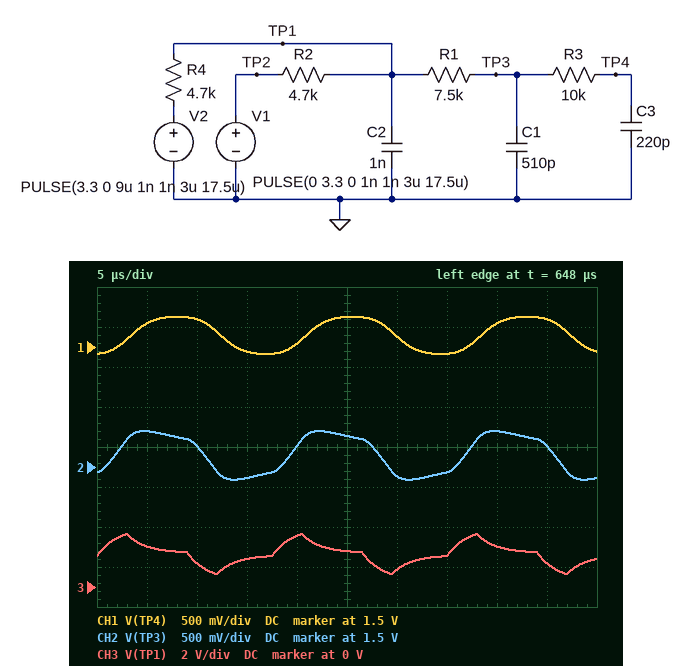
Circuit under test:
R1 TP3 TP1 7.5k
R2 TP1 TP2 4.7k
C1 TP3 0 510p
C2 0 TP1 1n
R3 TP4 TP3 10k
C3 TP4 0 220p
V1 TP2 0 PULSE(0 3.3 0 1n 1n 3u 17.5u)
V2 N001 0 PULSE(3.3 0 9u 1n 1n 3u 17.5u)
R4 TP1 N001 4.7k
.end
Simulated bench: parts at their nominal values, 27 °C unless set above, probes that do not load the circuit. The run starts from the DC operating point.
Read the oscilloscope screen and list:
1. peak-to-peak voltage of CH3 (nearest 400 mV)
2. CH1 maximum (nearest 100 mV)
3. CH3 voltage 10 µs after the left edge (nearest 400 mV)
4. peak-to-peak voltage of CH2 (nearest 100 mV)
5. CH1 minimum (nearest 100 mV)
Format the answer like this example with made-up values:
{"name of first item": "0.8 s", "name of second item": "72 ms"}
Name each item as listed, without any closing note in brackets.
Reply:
{"peak-to-peak voltage of CH3": "2.0 V", "CH1 maximum": "1.9 V", "CH3 voltage 10 µs after the left edge": "1.2 V", "peak-to-peak voltage of CH2": "600 mV", "CH1 minimum": "1.4 V"}
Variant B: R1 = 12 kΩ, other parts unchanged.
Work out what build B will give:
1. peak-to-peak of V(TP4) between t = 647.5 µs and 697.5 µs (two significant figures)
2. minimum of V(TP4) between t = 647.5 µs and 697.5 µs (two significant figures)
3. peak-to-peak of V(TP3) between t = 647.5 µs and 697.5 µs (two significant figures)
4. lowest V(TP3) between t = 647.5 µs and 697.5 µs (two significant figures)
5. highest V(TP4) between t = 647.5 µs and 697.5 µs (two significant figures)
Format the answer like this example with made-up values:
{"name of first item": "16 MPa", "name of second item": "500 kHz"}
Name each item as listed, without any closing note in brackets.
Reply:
{"peak-to-peak of V(TP4) between t = 647.5 µs and 697.5 µs": "340 mV", "minimum of V(TP4) between t = 647.5 µs and 697.5 µs": "1.5 V", "peak-to-peak of V(TP3) between t = 647.5 µs and 697.5 µs": "420 mV", "lowest V(TP3) between t = 647.5 µs and 697.5 µs": "1.4 V", "highest V(TP4) between t = 647.5 µs and 697.5 µs": "1.8 V"}
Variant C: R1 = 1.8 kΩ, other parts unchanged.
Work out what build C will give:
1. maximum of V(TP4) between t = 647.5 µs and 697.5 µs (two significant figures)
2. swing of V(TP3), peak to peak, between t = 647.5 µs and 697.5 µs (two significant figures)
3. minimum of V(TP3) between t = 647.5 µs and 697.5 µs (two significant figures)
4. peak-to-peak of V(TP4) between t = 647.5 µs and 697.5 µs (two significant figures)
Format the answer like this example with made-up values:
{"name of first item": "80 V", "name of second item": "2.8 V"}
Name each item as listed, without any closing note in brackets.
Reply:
{"maximum of V(TP4) between t = 647.5 µs and 697.5 µs": "2.0 V", "swing of V(TP3), peak to peak, between t = 647.5 µs and 697.5 µs": "1.2 V", "minimum of V(TP3) between t = 647.5 µs and 697.5 µs": "1.0 V", "peak-to-peak of V(TP4) between t = 647.5 µs and 697.5 µs": "790 mV"}
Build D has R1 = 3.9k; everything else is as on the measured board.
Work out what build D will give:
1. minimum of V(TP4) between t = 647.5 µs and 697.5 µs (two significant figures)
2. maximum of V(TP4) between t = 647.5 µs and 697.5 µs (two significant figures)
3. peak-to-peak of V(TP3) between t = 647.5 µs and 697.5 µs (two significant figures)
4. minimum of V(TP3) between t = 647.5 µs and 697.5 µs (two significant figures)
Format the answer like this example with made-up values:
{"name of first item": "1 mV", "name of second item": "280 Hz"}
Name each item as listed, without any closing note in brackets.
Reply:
{"minimum of V(TP4) between t = 647.5 µs and 697.5 µs": "1.3 V", "maximum of V(TP4) between t = 647.5 µs and 697.5 µs": "2.0 V", "peak-to-peak of V(TP3) between t = 647.5 µs and 697.5 µs": "910 mV", "minimum of V(TP3) between t = 647.5 µs and 697.5 µs": "1.2 V"}
